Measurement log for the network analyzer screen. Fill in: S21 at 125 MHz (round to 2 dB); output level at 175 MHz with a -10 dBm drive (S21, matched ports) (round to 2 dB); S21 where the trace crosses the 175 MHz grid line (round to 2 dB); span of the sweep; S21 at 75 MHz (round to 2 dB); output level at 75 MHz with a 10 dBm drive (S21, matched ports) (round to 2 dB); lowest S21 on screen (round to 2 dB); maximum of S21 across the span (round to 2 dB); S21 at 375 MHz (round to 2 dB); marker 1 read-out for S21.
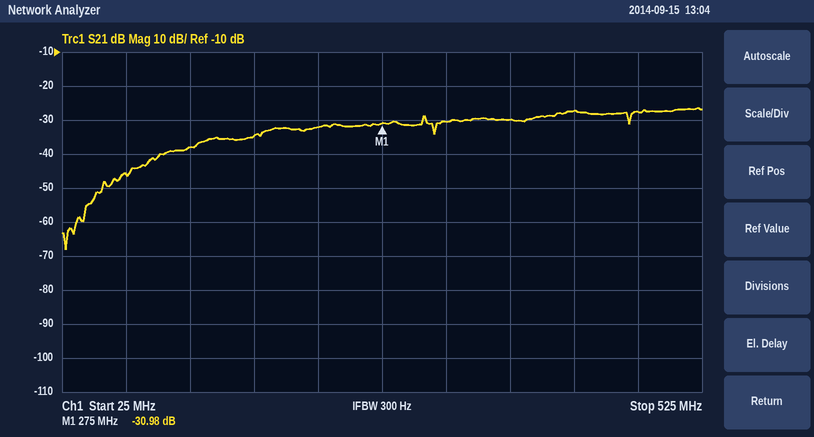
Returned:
-38 dB
-44 dBm
-34 dB
500 MHz
-46 dB
-36 dBm
-68 dB
-26 dB
-30 dB
-30.98 dB
